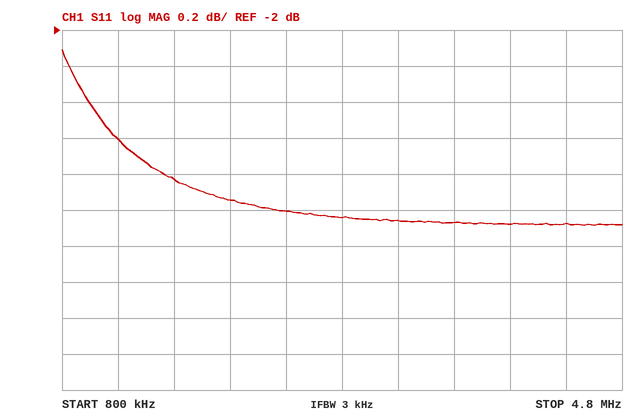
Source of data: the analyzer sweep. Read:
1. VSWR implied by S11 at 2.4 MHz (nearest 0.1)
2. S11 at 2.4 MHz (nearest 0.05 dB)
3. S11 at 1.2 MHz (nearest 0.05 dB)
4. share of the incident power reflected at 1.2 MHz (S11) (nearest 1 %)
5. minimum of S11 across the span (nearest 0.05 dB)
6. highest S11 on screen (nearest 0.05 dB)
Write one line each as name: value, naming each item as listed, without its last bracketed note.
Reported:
VSWR implied by S11 at 2.4 MHz: 5.8
S11 at 2.4 MHz: -3.00 dB
S11 at 1.2 MHz: -2.60 dB
share of the incident power reflected at 1.2 MHz (S11): 55 %
minimum of S11 across the span: -3.10 dB
highest S11 on screen: -2.10 dB
